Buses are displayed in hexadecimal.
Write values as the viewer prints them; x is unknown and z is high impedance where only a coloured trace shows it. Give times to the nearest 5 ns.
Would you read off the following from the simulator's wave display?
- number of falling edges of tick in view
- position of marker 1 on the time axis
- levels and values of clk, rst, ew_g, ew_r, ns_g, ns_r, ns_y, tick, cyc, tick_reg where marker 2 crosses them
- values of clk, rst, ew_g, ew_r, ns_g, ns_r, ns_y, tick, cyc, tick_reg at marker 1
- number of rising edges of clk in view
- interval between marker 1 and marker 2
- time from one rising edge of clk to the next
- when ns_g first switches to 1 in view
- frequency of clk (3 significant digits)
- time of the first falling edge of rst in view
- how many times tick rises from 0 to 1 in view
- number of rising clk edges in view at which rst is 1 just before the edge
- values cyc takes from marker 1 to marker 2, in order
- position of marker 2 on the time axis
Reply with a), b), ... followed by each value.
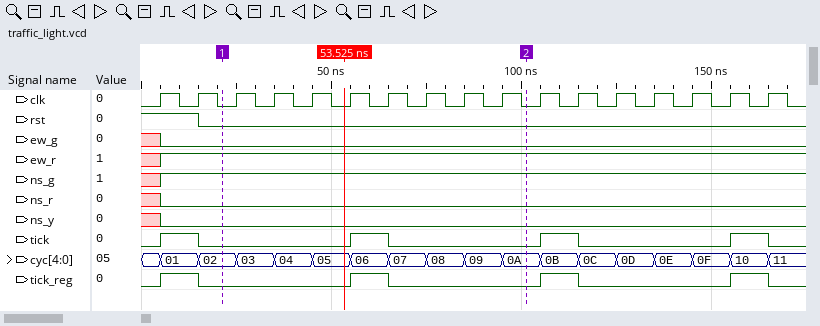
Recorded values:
a) 4
b) 20 ns
c) clk=0, rst=0, ew_g=0, ew_r=1, ns_g=1, ns_r=0, ns_y=0, tick=0, cyc=0A, tick_reg=0
d) clk=0, rst=0, ew_g=0, ew_r=1, ns_g=1, ns_r=0, ns_y=0, tick=0, cyc=02, tick_reg=0
e) 17
f) 80 ns
g) 10 ns
h) 5 ns
i) 100 MHz
j) 15 ns
k) 4
l) 2
m) 02, 03, 04, 05, 06, 07, 08, 09, 0A
n) 100 ns
